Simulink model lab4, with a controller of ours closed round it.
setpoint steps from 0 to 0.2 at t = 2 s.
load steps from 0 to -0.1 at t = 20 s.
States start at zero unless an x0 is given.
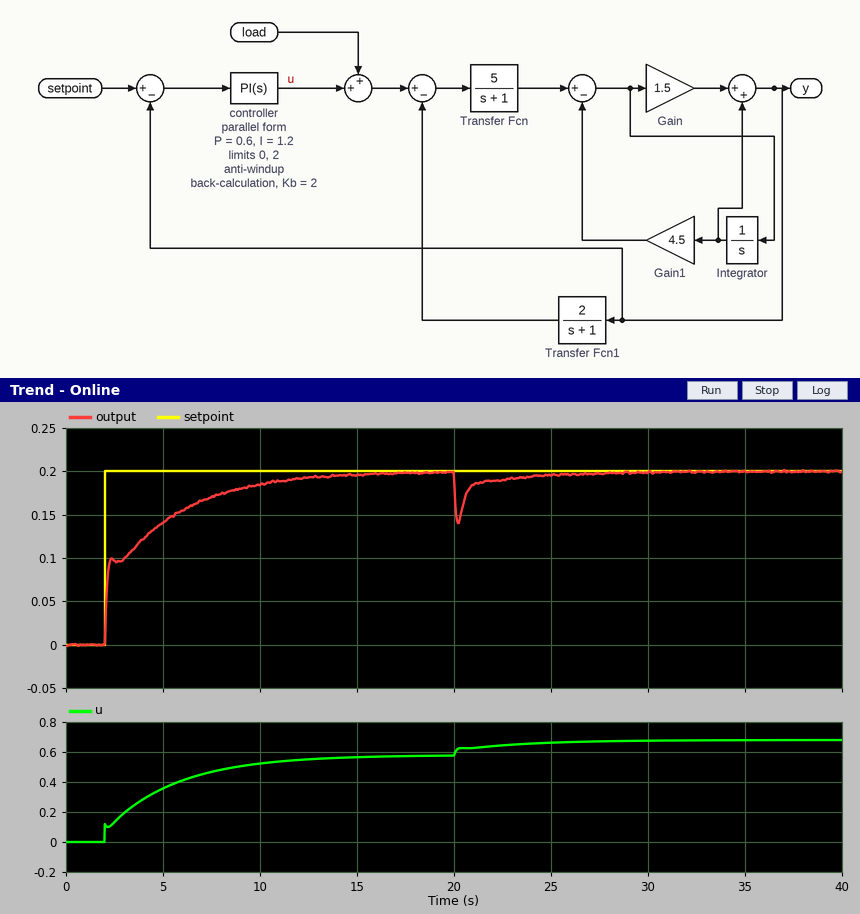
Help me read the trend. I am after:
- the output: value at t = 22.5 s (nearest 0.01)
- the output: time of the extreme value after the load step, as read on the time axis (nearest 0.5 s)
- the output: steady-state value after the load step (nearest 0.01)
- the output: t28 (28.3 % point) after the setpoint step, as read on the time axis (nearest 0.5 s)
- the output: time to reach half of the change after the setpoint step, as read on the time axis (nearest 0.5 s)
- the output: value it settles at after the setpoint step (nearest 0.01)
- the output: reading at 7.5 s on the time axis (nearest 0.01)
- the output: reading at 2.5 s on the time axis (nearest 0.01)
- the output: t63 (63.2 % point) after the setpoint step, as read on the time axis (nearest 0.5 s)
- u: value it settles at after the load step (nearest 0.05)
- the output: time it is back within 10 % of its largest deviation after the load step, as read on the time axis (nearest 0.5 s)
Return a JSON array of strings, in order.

["0.19", "20.0 s", "0.20", "2.0 s", "3.0 s", "0.20", "0.17", "0.10", "4.0 s", "0.70", "24.5 s"]
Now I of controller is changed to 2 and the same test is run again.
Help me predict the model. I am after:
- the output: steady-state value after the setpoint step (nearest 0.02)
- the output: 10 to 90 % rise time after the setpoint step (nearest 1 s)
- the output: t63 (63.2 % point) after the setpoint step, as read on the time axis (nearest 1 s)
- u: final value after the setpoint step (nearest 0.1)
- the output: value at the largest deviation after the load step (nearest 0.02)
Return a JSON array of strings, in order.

["0.20", "4 s", "3 s", "0.6", "0.14"]
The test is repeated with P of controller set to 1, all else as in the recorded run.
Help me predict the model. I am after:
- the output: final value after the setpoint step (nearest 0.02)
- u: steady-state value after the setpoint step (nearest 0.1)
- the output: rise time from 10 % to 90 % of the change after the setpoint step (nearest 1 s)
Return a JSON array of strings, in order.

["0.20", "0.6", "7 s"]
